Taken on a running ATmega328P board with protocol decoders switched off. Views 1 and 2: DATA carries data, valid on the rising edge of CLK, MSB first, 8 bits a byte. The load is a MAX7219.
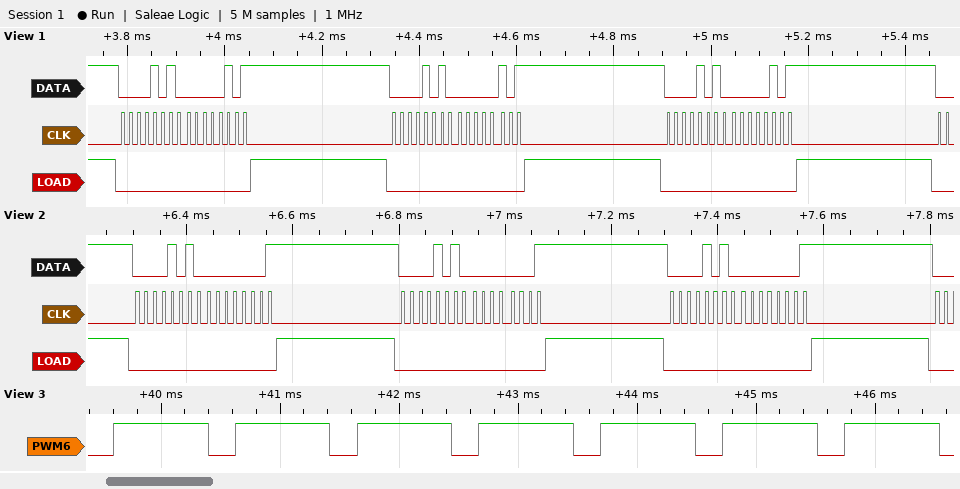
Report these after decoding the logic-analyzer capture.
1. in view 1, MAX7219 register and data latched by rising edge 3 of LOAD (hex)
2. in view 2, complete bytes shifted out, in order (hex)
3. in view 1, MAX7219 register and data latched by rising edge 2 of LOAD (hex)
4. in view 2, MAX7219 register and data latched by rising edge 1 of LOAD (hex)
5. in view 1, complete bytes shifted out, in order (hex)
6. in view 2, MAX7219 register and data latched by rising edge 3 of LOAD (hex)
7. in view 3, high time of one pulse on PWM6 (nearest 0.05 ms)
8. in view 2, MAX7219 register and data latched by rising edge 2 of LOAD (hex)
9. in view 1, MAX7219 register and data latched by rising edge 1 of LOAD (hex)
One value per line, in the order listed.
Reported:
register 0xA, data 0x05
0A 01 0A 01 0A 01
register 0xA, data 0x05
register 0xA, data 0x01
0A 05 0A 05 0A 05
register 0xA, data 0x01
0.80 ms
register 0xA, data 0x01
register 0xA, data 0x05
